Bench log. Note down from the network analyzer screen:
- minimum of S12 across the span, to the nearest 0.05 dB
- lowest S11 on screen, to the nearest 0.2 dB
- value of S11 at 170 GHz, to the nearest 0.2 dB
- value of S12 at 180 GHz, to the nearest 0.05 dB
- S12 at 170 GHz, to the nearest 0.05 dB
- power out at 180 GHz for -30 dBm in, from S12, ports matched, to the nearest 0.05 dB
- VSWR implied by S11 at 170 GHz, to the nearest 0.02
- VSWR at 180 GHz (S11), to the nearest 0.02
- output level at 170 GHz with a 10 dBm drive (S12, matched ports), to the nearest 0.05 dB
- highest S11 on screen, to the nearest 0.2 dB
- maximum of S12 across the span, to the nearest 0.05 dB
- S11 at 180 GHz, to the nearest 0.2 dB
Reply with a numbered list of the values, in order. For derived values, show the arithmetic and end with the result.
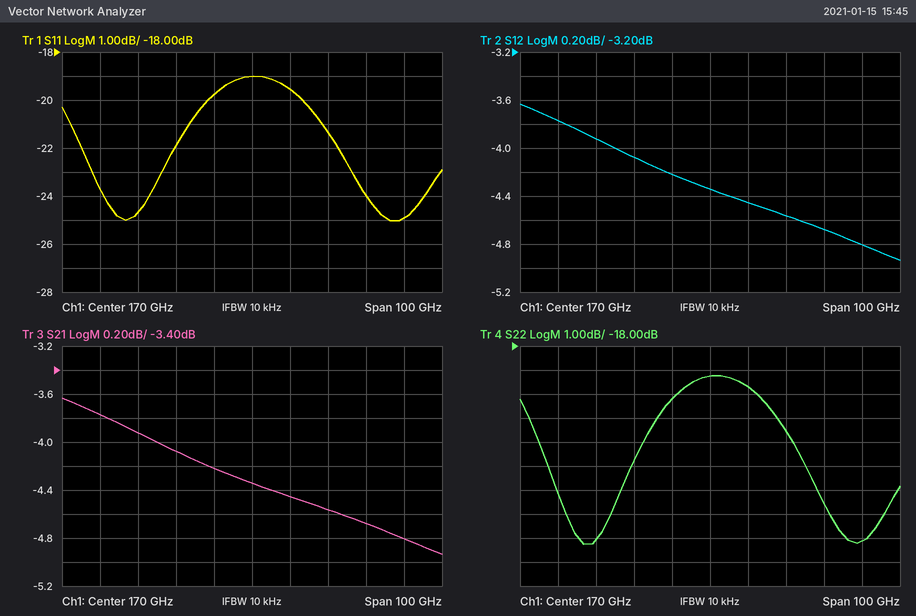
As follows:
1. -4.95 dB
2. -25.0 dB
3. -19.0 dB
4. -4.45 dB
5. -4.35 dB
6. -30 dBm + (-4.45 dB) = -34.45 dBm
7. |Γ| = 10^(-19/20) = 0.1122; VSWR = (1 + 0.1122)/(1 − 0.1122) ≈ 1.25, so 1.26 to the nearest 0.02
8. |Γ| = 10^(-19.6/20) = 0.1047; VSWR = (1 + 0.1047)/(1 − 0.1047) ≈ 1.23, so 1.24 to the nearest 0.02
9. 10 dBm + (-4.35 dB) = 5.65 dBm
10. -19.0 dB
11. -3.65 dB
12. -19.6 dB
